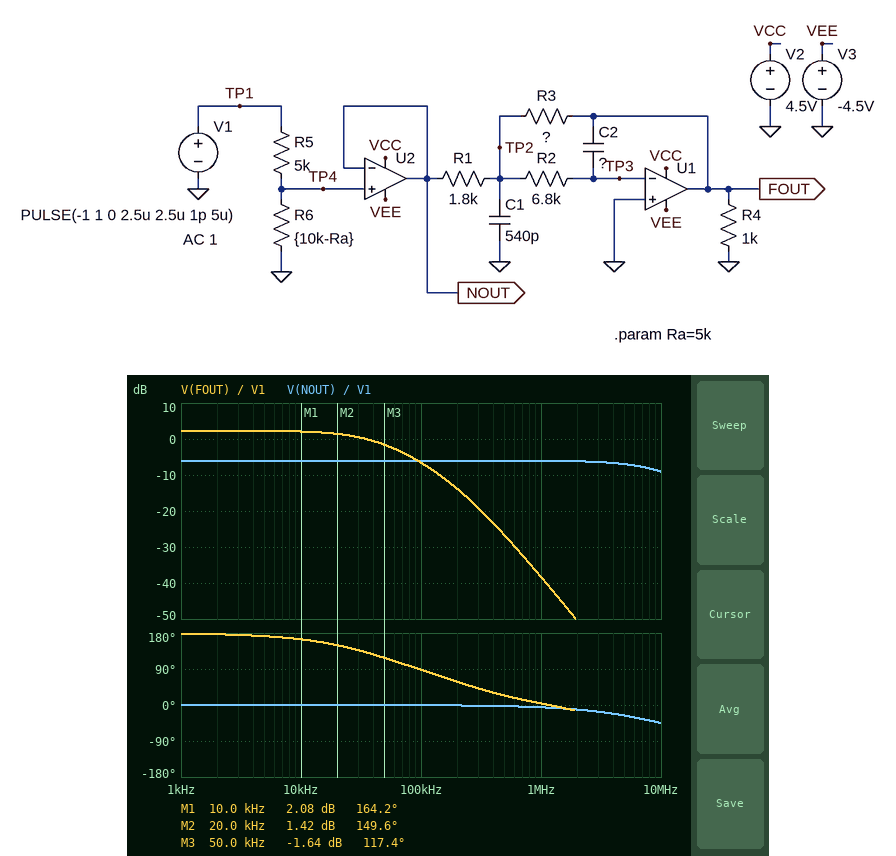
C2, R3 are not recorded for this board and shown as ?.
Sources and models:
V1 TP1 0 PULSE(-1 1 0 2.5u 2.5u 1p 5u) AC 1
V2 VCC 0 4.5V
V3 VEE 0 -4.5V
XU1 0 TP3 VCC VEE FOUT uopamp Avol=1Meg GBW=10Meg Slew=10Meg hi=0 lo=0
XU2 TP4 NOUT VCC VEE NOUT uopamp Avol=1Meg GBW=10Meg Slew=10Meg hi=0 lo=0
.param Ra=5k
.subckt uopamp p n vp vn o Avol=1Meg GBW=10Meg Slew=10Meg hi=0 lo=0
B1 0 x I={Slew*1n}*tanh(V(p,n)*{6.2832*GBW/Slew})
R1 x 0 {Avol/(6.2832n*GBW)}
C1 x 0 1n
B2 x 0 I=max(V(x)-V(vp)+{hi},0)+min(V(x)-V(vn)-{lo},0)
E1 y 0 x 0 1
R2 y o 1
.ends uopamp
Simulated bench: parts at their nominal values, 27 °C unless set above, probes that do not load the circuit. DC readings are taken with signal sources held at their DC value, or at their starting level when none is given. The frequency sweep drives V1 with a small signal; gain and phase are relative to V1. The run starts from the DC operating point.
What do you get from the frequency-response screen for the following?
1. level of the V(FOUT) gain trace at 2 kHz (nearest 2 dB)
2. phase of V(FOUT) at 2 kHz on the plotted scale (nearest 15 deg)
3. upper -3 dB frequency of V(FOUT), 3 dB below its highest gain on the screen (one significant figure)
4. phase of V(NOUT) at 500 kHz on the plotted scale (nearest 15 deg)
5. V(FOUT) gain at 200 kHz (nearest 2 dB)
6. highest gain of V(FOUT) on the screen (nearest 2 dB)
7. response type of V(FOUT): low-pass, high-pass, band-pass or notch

2 dB
180 deg
40 kHz
0 deg
-14 dB
2 dB
low-pass
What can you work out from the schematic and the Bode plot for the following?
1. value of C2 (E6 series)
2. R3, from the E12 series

150 pF
4.7 kΩ
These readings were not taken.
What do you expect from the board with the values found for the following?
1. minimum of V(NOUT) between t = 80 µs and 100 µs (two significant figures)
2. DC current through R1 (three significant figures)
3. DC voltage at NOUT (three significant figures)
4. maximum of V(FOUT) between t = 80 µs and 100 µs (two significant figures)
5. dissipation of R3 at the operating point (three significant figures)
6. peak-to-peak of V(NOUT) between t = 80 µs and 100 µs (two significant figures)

-500 mV
278 µA
-500 mV
160 mV
363 µW
990 mV
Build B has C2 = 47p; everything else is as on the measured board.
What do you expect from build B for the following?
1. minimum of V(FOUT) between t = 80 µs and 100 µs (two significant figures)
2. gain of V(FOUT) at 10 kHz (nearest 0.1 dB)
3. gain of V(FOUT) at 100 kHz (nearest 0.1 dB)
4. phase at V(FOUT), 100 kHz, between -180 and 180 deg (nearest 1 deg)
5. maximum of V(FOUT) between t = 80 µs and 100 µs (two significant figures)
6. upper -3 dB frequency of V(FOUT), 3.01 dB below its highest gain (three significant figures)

-580 mV
2.3 dB
1.4 dB
126 deg
580 mV
158 kHz
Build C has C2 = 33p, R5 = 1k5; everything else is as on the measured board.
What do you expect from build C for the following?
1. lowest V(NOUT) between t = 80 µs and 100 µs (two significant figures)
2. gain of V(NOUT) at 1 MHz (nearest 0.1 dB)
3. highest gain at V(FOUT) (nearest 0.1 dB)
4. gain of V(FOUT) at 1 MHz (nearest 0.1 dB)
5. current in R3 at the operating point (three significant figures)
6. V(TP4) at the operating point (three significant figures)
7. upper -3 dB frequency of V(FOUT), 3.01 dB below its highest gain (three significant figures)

-760 mV
-2.3 dB
6.2 dB
-21.6 dB
427 µA
-769 mV
219 kHz
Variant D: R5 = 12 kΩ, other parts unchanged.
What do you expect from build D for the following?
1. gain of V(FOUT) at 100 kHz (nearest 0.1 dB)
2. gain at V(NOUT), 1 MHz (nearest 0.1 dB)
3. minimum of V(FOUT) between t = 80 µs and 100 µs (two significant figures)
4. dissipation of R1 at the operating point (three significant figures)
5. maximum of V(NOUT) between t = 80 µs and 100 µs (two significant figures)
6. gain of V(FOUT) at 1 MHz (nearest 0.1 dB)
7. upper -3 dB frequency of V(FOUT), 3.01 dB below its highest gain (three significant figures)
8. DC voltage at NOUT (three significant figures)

-11.2 dB
-10.7 dB
-96 mV
48.1 µW
290 mV
-42.9 dB
41.3 kHz
-294 mV
